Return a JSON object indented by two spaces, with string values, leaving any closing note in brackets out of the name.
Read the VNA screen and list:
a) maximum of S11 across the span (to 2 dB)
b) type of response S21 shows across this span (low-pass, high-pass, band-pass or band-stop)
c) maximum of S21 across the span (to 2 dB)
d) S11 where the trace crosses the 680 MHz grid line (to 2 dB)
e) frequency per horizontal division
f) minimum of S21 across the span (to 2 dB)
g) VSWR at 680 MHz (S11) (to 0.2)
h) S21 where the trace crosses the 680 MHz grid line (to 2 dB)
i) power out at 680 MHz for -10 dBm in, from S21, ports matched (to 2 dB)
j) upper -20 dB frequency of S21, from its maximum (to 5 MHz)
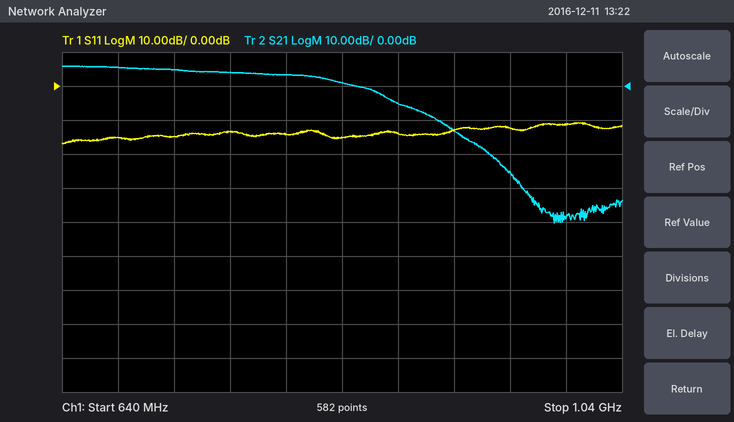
{
  "maximum of S11 across the span": "-10 dB",
  "type of response S21 shows across this span": "low-pass",
  "maximum of S21 across the span": "6 dB",
  "S11 where the trace crosses the 680 MHz grid line": "-16 dB",
  "frequency per horizontal division": "40 MHz",
  "minimum of S21 across the span": "-40 dB",
  "VSWR at 680 MHz (S11)": "1.4",
  "S21 where the trace crosses the 680 MHz grid line": "6 dB",
  "power out at 680 MHz for -10 dBm in, from S21, ports matched": "-4 dBm",
  "upper -20 dB frequency of S21, from its maximum": "925 MHz"
}
